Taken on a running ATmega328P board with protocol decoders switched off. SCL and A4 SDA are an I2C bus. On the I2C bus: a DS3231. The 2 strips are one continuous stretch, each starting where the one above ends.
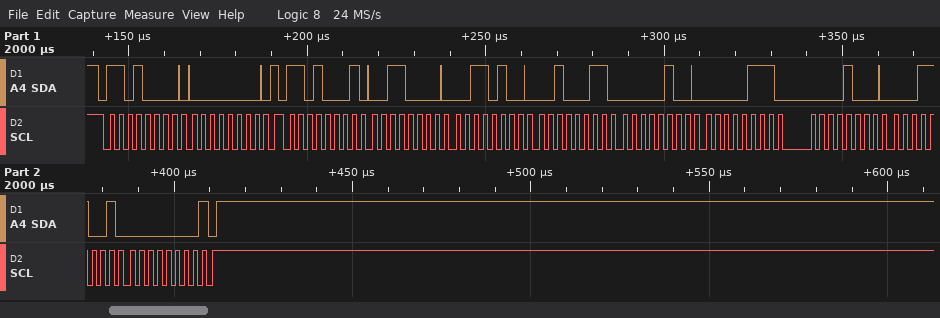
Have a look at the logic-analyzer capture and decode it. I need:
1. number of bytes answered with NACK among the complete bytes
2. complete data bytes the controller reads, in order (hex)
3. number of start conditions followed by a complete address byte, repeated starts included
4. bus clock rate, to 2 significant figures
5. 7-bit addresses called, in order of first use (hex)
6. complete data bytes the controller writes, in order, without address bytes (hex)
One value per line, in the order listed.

1
30 34 23 04 07 08 19 00
2
400 kHz
0x68
00
